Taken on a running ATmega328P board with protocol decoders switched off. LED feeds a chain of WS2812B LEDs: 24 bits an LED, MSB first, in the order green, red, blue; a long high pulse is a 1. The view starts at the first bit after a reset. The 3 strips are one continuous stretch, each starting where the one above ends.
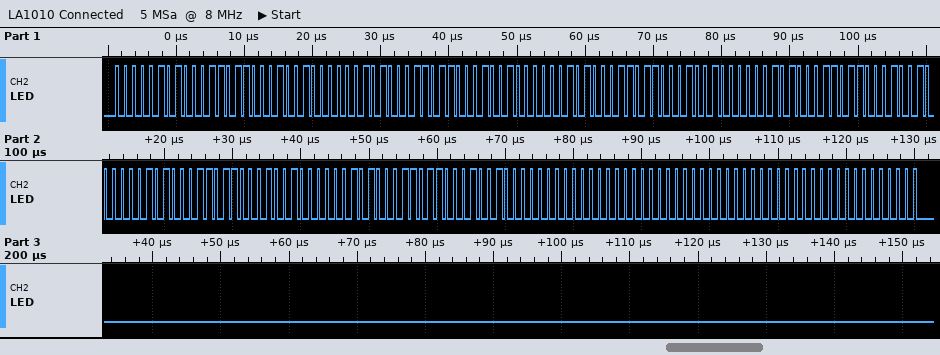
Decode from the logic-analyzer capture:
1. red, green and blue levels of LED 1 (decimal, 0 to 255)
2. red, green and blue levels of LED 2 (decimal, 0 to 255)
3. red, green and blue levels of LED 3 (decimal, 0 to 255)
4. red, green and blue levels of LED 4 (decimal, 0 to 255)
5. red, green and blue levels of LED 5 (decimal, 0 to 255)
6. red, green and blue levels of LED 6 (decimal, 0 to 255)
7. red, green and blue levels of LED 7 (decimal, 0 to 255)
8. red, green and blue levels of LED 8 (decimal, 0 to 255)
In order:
27, 5, 18
27, 5, 18
27, 5, 18
27, 5, 18
27, 5, 18
27, 5, 18
0, 0, 0
0, 0, 0
